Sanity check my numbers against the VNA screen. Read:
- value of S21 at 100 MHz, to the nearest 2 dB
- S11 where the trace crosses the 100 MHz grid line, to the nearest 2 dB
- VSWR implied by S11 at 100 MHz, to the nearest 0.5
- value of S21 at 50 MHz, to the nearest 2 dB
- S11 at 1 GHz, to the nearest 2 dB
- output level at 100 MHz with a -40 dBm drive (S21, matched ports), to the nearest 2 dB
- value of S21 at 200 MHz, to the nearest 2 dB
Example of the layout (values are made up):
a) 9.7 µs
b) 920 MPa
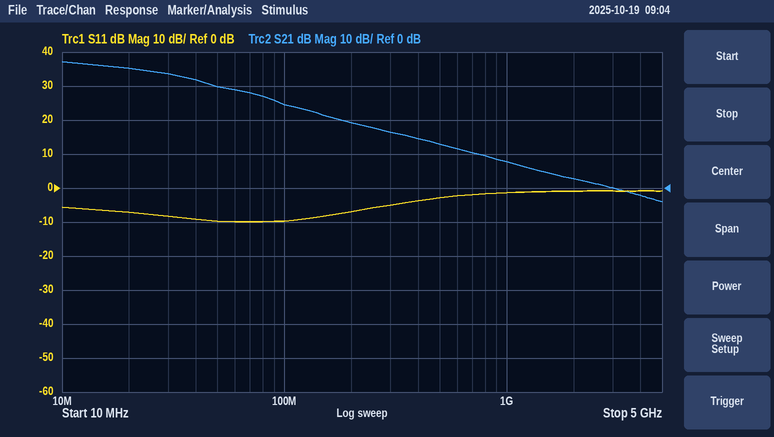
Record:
a) 24 dB
b) -10 dB
c) 2.0
d) 30 dB
e) -2 dB
f) -16 dBm
g) 20 dB
